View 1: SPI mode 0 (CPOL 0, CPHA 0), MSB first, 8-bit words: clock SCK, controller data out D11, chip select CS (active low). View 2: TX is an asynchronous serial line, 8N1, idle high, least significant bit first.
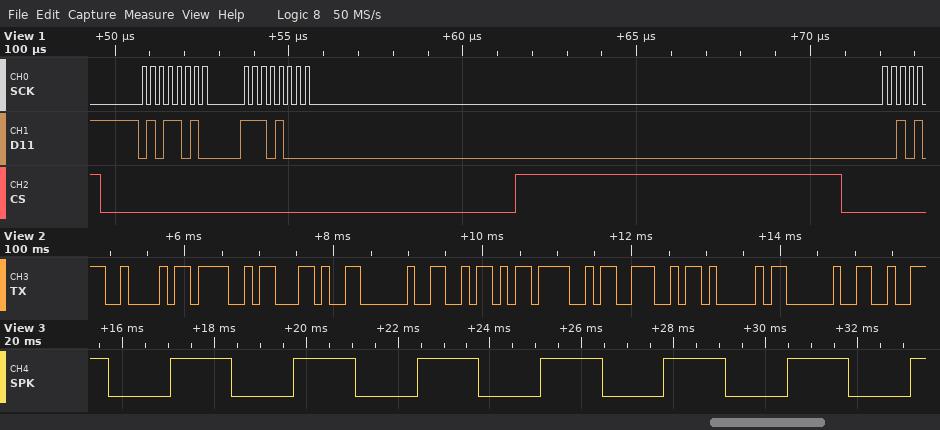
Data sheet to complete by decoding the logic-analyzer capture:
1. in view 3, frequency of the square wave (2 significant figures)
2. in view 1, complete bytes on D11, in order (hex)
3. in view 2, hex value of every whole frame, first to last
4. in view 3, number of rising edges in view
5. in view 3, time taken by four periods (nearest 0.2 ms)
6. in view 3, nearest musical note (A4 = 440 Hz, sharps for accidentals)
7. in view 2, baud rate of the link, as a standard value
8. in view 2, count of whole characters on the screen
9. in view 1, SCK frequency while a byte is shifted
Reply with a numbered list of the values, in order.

1. 370 Hz
2. 0x5A 0xE8
3. 42 4F 2C 20 5A 4F 4E 41 20
4. 7
5. 10.8 ms
6. F#4
7. 9600 baud
8. 9
9. 4 MHz
